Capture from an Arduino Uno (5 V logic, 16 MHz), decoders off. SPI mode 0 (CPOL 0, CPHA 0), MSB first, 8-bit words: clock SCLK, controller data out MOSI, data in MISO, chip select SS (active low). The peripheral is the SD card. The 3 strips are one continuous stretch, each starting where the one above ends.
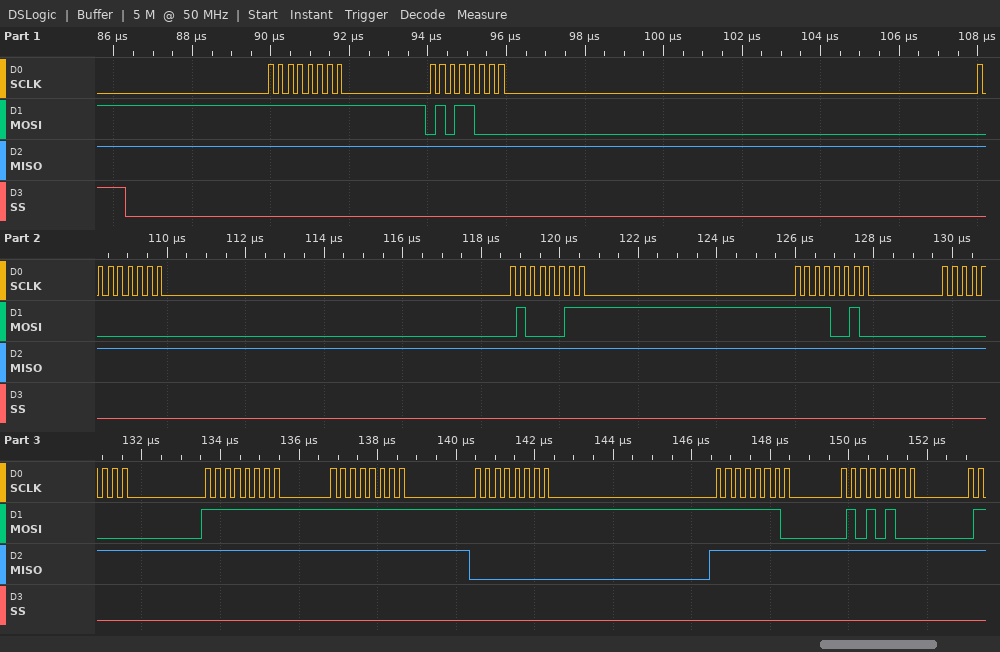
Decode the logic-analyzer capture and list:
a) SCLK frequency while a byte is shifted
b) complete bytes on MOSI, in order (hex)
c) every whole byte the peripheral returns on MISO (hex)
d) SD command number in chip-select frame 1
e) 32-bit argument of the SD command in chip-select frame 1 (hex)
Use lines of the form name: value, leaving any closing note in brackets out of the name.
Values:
SCLK frequency while a byte is shifted: 4 MHz
complete bytes on MOSI, in order: 0xFF 0x58 0x00 0x43 0xF2 0x00 0xFF 0xFF 0xFF 0xFE 0x54
every whole byte the peripheral returns on MISO: 0xFF 0xFF 0xFF 0xFF 0xFF 0xFF 0xFF 0xFF 0x00 0xFF 0xFF
SD command number in chip-select frame 1: CMD24
32-bit argument of the SD command in chip-select frame 1: 0x0043F200
